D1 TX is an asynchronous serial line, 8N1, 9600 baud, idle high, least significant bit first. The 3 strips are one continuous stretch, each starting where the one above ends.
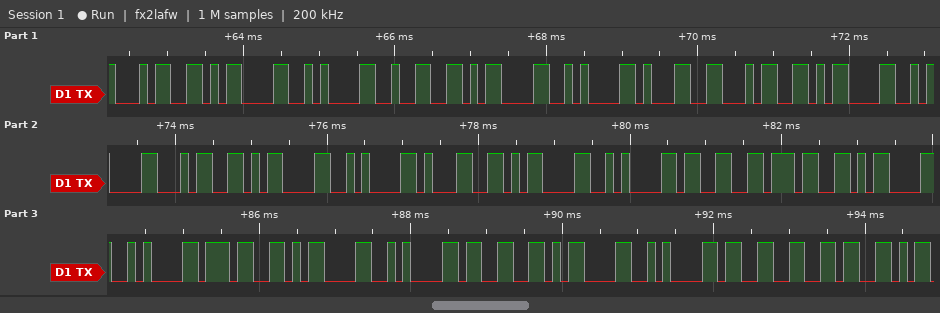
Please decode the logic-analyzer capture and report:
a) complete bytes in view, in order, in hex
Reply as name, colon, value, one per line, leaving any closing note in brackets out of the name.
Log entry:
complete bytes in view, in order, in hex: 34 0D 0A 32 0D 0A 31 34 0D 0A 34 0D 0A 31 0D 0A 33 37 0D 0A 37 0D 0A 33 0D 0A 33 36
